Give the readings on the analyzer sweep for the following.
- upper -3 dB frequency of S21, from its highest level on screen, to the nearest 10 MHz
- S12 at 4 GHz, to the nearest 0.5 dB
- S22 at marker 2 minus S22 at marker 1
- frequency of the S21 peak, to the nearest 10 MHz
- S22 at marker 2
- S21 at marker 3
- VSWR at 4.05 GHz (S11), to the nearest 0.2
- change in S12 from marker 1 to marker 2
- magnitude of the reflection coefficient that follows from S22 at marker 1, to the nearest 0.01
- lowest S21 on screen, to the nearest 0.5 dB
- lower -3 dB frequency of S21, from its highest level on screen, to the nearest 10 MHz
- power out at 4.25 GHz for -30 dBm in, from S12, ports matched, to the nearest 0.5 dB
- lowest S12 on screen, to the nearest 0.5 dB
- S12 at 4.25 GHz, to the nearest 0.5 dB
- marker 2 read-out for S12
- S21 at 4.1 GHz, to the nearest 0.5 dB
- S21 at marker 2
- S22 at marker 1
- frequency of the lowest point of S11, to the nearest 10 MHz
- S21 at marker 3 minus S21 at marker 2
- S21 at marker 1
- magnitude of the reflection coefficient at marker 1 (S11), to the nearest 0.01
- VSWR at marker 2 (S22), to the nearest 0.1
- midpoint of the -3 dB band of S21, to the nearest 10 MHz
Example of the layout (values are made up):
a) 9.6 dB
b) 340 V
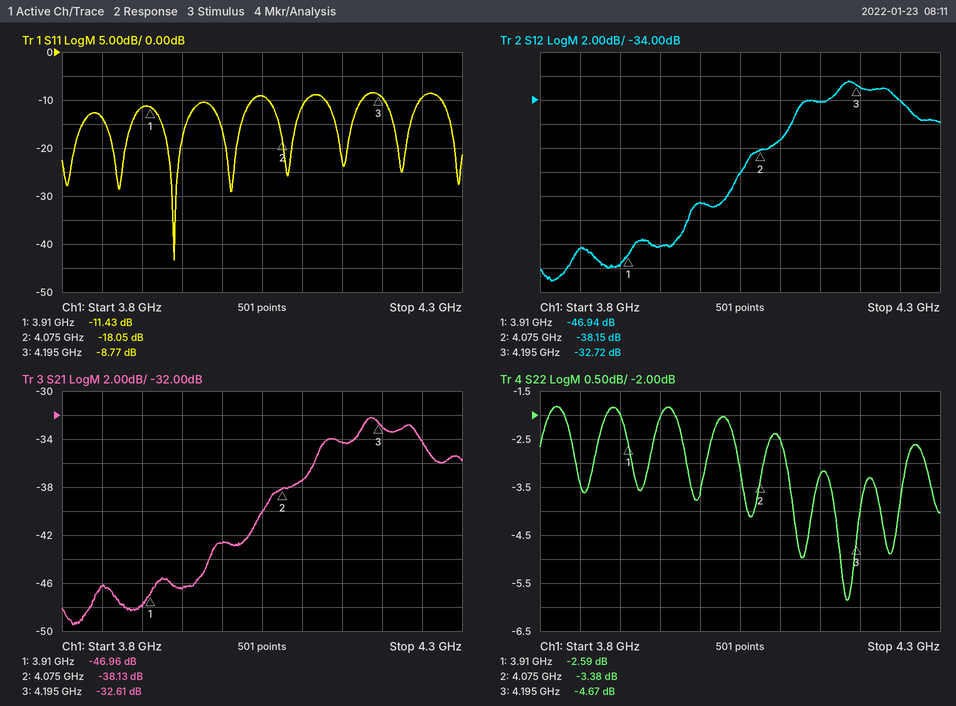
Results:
a) 4.26 GHz
b) -42.5 dB
c) -0.79 dB
d) 4.19 GHz
e) -3.38 dB
f) -32.61 dB
g) 2.0
h) 8.79 dB
i) 0.74
j) -49.5 dB
k) 4.12 GHz
l) -64.0 dBm
m) -49.0 dB
n) -34.0 dB
o) -38.15 dB
p) -37.5 dB
q) -38.13 dB
r) -2.59 dB
s) 3.94 GHz
t) 5.52 dB
u) -46.96 dB
v) 0.27
w) 5.2
x) 4.19 GHz
